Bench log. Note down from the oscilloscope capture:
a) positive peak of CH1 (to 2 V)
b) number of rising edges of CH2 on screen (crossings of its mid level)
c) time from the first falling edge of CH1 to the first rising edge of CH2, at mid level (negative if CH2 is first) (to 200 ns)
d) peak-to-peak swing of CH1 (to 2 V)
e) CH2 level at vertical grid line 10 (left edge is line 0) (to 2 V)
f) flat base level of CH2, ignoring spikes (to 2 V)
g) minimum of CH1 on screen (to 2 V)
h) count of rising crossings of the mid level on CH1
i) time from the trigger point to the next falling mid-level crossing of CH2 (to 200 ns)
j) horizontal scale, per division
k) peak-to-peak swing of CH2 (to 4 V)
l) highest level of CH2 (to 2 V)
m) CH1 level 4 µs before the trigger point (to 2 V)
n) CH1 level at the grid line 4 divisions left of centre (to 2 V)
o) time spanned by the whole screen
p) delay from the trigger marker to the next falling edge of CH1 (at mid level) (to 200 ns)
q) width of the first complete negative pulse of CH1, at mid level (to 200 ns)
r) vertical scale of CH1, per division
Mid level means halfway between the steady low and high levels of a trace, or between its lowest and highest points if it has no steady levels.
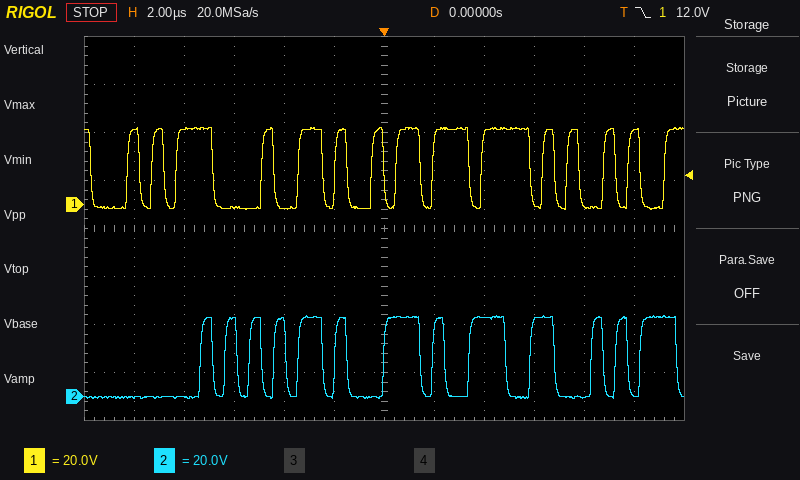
32 V
13
+4.4 µs
34 V
0 V
0 V
-2 V
15
1.4 µs
2 µs
36 V
34 V
-2 V
32 V
24 µs
1.4 µs
1.4 µs
20 V
